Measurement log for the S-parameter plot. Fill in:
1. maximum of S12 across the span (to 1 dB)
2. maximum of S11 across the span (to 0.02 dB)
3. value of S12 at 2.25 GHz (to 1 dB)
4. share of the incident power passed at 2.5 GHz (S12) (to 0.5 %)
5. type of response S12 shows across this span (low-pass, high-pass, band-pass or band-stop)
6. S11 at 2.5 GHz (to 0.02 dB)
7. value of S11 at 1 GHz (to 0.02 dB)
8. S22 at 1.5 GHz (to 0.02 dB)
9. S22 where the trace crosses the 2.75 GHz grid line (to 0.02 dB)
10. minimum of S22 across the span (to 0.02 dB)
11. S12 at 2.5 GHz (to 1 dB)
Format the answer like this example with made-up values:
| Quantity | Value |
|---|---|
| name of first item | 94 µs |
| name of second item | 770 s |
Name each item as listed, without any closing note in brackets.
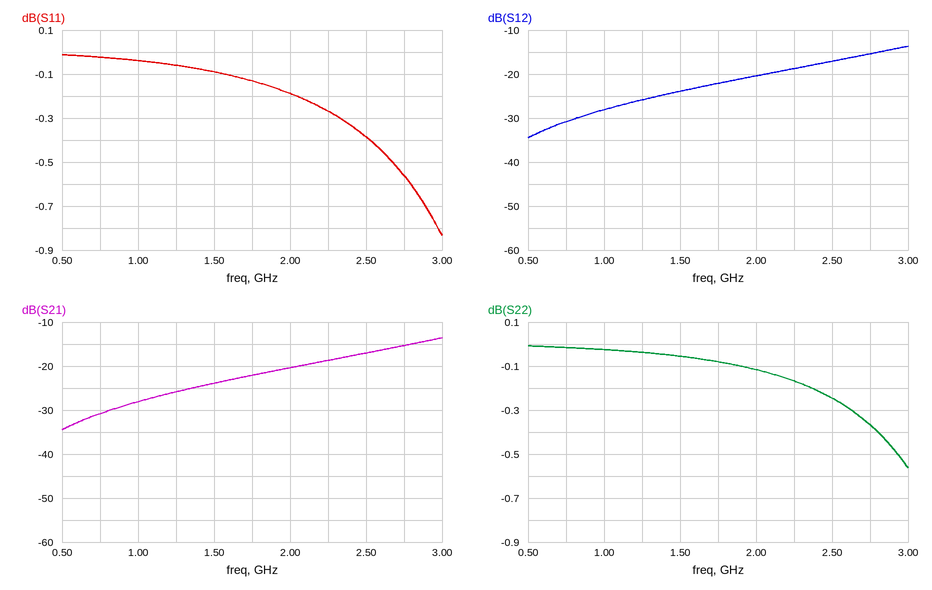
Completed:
| Quantity | Value |
|---|---|
| maximum of S12 across the span | -14 dB |
| maximum of S11 across the span | -0.02 dB |
| value of S12 at 2.25 GHz | -19 dB |
| share of the incident power passed at 2.5 GHz (S12) | 2.0 % |
| type of response S12 shows across this span | high-pass |
| S11 at 2.5 GHz | -0.38 dB |
| value of S11 at 1 GHz | -0.04 dB |
| S22 at 1.5 GHz | -0.06 dB |
| S22 where the trace crosses the 2.75 GHz grid line | -0.36 dB |
| minimum of S22 across the span | -0.56 dB |
| S12 at 2.5 GHz | -17 dB |
